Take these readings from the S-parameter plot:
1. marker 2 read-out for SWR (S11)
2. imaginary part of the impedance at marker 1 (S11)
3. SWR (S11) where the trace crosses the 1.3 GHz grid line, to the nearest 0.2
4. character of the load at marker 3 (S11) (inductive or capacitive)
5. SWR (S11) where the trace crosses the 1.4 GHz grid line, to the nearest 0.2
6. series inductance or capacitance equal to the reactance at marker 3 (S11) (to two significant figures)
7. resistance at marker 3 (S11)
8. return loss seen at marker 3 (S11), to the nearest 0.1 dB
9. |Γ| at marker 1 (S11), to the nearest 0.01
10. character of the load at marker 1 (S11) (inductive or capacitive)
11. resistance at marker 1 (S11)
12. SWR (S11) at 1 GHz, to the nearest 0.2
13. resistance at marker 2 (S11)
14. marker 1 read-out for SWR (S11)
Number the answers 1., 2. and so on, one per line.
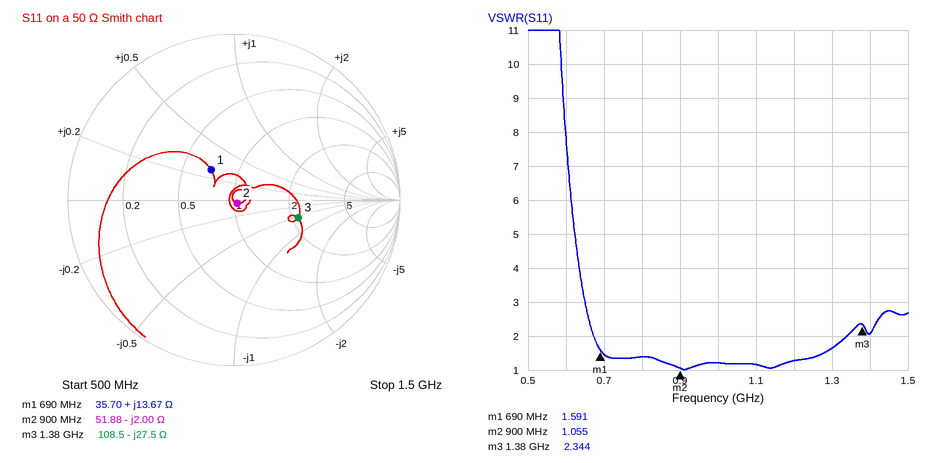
1. 1.055
2. +13.67 Ω
3. 1.6
4. capacitive
5. 2.0
6. 4.2 pF
7. 108.5 Ω
8. 7.9 dB
9. 0.23
10. inductive
11. 35.70 Ω
12. 1.2
13. 51.88 Ω
14. 1.591
